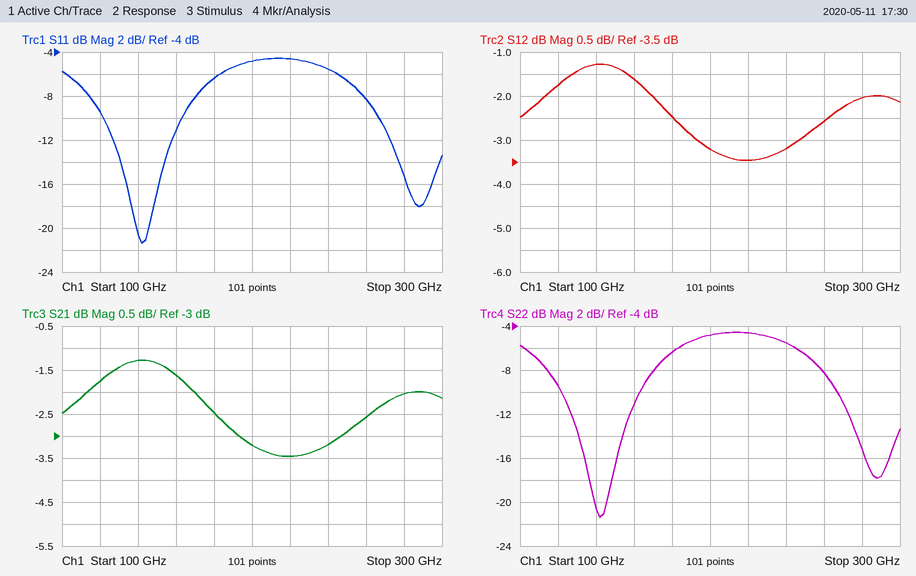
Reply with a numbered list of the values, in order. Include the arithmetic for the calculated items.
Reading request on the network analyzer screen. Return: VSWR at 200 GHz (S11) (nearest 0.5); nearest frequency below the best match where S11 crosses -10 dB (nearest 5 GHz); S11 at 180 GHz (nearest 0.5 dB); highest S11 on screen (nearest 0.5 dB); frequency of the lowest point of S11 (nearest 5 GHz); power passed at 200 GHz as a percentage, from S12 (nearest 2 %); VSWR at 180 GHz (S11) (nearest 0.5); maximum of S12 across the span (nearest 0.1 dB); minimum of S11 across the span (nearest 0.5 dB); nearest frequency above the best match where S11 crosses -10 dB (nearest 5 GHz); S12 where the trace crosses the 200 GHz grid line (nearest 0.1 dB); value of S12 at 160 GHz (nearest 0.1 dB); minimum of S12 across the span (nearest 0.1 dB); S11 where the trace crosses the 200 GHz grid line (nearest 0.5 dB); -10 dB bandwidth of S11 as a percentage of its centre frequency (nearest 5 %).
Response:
1. |Γ| = 10^(-5/20) = 0.5623; VSWR = (1 + 0.5623)/(1 − 0.5623) ≈ 3.57, so 3.5 to the nearest 0.5
2. 120 GHz
3. -6.5 dB
4. -4.5 dB
5. 140 GHz
6. 10^(-3.2/10) ≈ 48 %
7. |Γ| = 10^(-6.5/20) = 0.4732; VSWR = (1 + 0.4732)/(1 − 0.4732) ≈ 2.80, so 3.0 to the nearest 0.5
8. -1.3 dB
9. -21.5 dB
10. 165 GHz
11. -3.2 dB
12. -1.6 dB
13. -3.5 dB
14. -5.0 dB
15. 45 GHz / 142.5 GHz ≈ 31.6 %, so 30 % to the nearest 5 %
